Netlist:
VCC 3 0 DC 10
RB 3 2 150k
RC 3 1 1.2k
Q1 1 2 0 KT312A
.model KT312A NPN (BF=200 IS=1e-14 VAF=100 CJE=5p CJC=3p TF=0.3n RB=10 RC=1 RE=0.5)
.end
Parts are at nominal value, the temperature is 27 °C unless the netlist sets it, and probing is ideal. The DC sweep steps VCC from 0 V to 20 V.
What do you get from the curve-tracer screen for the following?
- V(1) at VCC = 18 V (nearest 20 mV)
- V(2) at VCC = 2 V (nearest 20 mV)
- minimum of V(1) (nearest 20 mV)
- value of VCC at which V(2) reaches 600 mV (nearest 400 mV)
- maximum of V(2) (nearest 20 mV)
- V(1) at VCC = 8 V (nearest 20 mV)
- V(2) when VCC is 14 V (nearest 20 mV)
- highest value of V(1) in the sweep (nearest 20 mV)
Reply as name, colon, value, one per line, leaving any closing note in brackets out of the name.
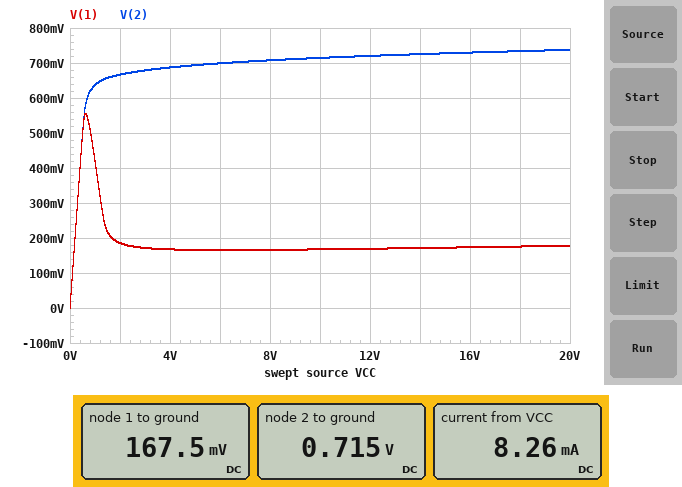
V(1) at VCC = 18 V: 180 mV
V(2) at VCC = 2 V: 660 mV
minimum of V(1): 0 V
value of VCC at which V(2) reaches 600 mV: 800 mV
maximum of V(2): 740 mV
V(1) at VCC = 8 V: 160 mV
V(2) when VCC is 14 V: 720 mV
highest value of V(1) in the sweep: 560 mV
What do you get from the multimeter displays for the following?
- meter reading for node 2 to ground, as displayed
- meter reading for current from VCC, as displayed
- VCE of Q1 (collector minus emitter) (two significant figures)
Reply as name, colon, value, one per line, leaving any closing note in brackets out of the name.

meter reading for node 2 to ground, as displayed: 0.715 V
meter reading for current from VCC, as displayed: 8.26 mA
VCE of Q1 (collector minus emitter): 170 mV
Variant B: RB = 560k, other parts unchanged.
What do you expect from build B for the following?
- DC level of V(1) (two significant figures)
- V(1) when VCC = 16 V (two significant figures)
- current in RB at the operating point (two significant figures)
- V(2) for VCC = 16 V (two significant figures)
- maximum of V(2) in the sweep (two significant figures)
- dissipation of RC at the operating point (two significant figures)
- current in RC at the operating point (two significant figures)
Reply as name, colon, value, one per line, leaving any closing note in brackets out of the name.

DC level of V(1): 5.8 V
V(1) when VCC = 16 V: 8.9 V
current in RB at the operating point: 17 µA
V(2) for VCC = 16 V: 700 mV
maximum of V(2) in the sweep: 710 mV
dissipation of RC at the operating point: 15 mW
current in RC at the operating point: 3.5 mA
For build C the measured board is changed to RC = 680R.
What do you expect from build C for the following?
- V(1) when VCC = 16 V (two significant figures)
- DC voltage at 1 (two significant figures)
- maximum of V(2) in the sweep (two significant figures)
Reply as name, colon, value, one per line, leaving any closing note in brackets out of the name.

V(1) when VCC = 16 V: 2.0 V
DC voltage at 1: 1.5 V
maximum of V(2) in the sweep: 750 mV
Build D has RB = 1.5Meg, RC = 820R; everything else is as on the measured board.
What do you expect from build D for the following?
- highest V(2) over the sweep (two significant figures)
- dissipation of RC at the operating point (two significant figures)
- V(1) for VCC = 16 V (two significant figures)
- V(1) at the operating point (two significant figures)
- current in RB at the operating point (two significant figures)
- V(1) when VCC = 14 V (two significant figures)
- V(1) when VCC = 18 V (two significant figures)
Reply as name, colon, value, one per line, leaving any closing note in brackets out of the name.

highest V(2) over the sweep: 680 mV
dissipation of RC at the operating point: 1.5 mW
V(1) for VCC = 16 V: 14 V
V(1) at the operating point: 8.9 V
current in RB at the operating point: 6.2 µA
V(1) when VCC = 14 V: 12 V
V(1) when VCC = 18 V: 16 V
